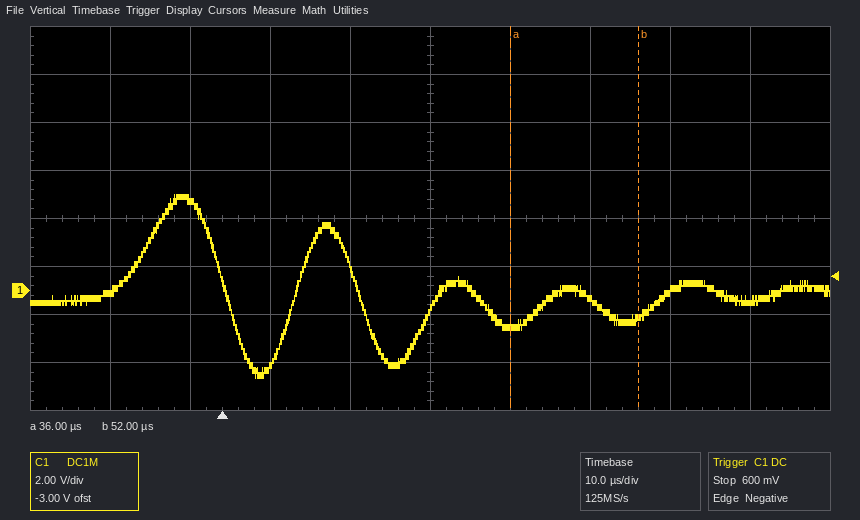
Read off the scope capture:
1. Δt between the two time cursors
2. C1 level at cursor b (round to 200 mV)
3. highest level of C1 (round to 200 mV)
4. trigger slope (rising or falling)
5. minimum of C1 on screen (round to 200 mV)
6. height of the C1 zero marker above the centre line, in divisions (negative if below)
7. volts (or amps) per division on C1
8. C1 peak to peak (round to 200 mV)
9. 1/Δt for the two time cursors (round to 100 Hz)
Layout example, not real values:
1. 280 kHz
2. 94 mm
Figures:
1. 16 µs
2. -1.2 V
3. 4.0 V
4. falling
5. -3.6 V
6. -1.5 div
7. 2 V
8. 7.6 V
9. 62.5 kHz
